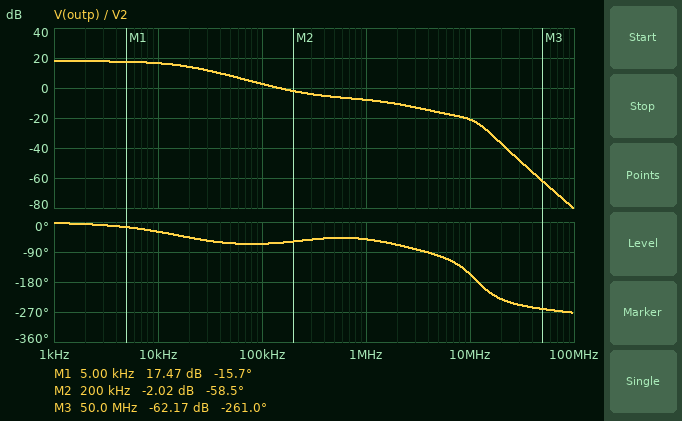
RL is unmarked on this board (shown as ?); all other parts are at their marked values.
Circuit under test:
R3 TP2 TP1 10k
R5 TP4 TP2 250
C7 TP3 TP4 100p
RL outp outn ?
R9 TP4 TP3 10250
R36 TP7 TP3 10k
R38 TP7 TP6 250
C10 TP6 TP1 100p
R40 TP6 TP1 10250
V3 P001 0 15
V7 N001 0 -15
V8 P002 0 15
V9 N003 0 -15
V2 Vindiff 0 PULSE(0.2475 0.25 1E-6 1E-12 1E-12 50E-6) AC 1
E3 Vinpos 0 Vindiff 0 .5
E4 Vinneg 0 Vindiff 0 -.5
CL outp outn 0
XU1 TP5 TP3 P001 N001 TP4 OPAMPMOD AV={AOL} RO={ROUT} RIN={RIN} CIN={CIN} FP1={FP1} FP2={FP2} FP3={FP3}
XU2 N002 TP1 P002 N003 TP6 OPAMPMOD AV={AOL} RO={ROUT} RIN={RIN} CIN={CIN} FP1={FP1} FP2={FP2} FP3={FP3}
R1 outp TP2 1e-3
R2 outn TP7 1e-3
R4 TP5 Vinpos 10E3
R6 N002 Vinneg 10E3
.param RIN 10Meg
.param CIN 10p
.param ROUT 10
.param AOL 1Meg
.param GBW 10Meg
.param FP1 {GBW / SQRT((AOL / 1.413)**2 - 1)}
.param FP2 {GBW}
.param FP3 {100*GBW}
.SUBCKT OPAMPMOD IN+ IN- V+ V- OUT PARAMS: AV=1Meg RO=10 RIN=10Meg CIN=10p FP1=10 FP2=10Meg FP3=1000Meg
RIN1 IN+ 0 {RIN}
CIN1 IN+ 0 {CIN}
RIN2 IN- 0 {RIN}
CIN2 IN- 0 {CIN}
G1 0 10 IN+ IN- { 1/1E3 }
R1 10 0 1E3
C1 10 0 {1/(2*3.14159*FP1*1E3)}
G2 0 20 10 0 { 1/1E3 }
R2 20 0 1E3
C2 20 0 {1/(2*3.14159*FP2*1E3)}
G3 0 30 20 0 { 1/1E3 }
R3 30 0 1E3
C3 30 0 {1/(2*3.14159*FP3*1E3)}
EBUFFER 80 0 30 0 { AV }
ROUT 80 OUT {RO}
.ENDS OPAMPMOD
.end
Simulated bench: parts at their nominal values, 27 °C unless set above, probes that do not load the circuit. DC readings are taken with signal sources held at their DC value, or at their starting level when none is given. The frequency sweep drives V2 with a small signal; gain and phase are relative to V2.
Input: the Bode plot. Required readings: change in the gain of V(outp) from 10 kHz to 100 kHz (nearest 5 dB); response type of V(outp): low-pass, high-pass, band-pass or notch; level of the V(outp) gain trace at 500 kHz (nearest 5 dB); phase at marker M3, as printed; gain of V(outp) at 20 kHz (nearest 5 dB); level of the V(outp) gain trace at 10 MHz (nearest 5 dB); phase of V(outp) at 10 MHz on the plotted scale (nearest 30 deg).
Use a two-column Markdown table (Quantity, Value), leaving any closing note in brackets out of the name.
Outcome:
| Quantity | Value |
|---|---|
| change in the gain of V(outp) from 10 kHz to 100 kHz | -15 dB |
| response type of V(outp): low-pass, high-pass, band-pass or notch | low-pass |
| level of the V(outp) gain trace at 500 kHz | -5 dB |
| phase at marker M3, as printed | -261.0 deg |
| gain of V(outp) at 20 kHz | 15 dB |
| level of the V(outp) gain trace at 10 MHz | -20 dB |
| phase of V(outp) at 10 MHz on the plotted scale | -150 deg |
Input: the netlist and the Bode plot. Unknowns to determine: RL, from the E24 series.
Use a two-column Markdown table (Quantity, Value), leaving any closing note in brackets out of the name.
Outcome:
| Quantity | Value |
|---|---|
| RL, from the E24 series | 3.9 kΩ |
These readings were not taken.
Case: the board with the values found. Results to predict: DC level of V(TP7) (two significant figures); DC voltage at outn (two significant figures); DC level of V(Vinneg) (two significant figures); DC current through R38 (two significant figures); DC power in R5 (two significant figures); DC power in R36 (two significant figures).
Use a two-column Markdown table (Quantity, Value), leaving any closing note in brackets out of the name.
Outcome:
| Quantity | Value |
|---|---|
| DC level of V(TP7) | -1.9 V |
| DC voltage at outn | -1.9 V |
| DC level of V(Vinneg) | -120 mV |
| DC current through R38 | 1.2 mA |
| DC power in R5 | 360 µW |
| DC power in R36 | 420 µW |
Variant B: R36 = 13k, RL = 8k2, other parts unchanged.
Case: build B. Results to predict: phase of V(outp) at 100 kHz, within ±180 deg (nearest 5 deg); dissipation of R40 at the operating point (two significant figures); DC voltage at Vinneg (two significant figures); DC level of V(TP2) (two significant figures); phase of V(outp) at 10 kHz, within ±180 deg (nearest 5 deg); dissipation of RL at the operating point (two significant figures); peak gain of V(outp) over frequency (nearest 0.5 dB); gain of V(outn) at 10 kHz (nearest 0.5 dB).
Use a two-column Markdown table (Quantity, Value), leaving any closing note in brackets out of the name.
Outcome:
| Quantity | Value |
|---|---|
| phase of V(outp) at 100 kHz, within ±180 deg | -60 deg |
| dissipation of R40 at the operating point | 170 µW |
| DC voltage at Vinneg | -120 mV |
| DC level of V(TP2) | 1.2 V |
| phase of V(outp) at 10 kHz, within ±180 deg | -20 deg |
| dissipation of RL at the operating point | 780 µW |
| peak gain of V(outp) over frequency | 13.5 dB |
| gain of V(outn) at 10 kHz | 14.0 dB |
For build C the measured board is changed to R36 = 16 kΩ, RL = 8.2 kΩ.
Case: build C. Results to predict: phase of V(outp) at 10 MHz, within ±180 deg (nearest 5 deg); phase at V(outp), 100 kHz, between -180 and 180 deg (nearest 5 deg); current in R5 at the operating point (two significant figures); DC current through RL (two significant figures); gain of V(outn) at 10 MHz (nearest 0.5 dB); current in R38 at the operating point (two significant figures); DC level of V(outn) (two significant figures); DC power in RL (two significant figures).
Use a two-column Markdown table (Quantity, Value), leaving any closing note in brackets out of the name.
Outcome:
| Quantity | Value |
|---|---|
| phase of V(outp) at 10 MHz, within ±180 deg | -155 deg |
| phase at V(outp), 100 kHz, between -180 and 180 deg | -50 deg |
| current in R5 at the operating point | 290 µA |
| DC current through RL | 200 µA |
| gain of V(outn) at 10 MHz | -20.5 dB |
| current in R38 at the operating point | 270 µA |
| DC level of V(outn) | -930 mV |
| DC power in RL | 330 µW |
